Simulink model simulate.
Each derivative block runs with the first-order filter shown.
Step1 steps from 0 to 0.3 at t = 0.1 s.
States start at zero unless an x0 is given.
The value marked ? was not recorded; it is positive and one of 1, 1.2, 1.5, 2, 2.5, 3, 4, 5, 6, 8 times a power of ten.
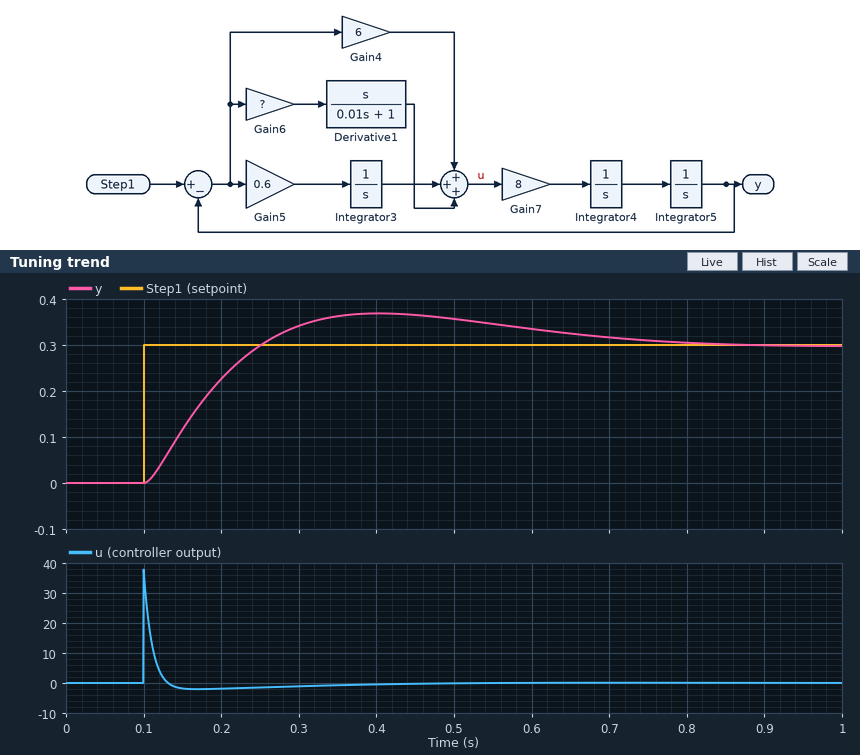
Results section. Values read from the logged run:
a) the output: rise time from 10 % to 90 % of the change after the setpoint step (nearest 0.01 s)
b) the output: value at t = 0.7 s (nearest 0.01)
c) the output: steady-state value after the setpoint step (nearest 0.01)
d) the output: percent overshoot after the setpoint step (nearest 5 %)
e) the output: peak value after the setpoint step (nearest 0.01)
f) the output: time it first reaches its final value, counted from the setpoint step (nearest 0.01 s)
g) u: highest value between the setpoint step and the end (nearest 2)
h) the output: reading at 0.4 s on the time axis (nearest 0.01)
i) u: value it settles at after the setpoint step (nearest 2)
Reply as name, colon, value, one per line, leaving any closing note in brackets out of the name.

the output: rise time from 10 % to 90 % of the change after the setpoint step: 0.11 s
the output: value at t = 0.7 s: 0.32
the output: steady-state value after the setpoint step: 0.30
the output: percent overshoot after the setpoint step: 25 %
the output: peak value after the setpoint step: 0.37
the output: time it first reaches its final value, counted from the setpoint step: 0.15 s
u: highest value between the setpoint step and the end: 38
the output: reading at 0.4 s on the time axis: 0.37
u: value it settles at after the setpoint step: 0
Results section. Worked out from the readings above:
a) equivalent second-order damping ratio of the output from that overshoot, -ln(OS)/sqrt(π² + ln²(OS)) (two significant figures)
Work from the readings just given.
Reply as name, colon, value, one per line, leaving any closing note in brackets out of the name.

equivalent second-order damping ratio of the output from that overshoot, -ln(OS)/sqrt(π² + ln²(OS)): 0.40
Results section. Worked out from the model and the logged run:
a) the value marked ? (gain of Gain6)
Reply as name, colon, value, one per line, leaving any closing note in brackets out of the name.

the value marked ?: 1.2
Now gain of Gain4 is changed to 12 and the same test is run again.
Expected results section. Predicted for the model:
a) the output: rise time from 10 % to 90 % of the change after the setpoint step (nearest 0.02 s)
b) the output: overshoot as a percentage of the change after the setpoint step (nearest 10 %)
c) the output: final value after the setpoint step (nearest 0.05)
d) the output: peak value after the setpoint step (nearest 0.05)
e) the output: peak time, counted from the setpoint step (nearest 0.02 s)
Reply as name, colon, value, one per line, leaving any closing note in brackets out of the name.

the output: rise time from 10 % to 90 % of the change after the setpoint step: 0.08 s
the output: overshoot as a percentage of the change after the setpoint step: 30 %
the output: final value after the setpoint step: 0.30
the output: peak value after the setpoint step: 0.40
the output: peak time, counted from the setpoint step: 0.24 s
